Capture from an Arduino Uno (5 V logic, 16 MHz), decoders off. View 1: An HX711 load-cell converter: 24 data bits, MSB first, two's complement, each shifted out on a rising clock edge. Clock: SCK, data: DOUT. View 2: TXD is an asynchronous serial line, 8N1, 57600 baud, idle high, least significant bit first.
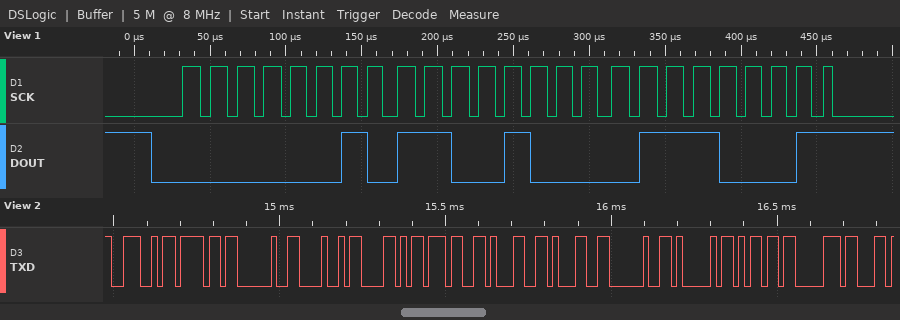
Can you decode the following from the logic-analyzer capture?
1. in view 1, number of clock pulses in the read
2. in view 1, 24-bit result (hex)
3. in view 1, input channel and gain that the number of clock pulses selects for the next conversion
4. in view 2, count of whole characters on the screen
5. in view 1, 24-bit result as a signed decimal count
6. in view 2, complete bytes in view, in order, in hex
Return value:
25
0x02C871
channel A, gain 128
12
182385
0x4E 0x6F 0x20 0x48 0x58 0x37 0x31 0x31 0x20 0x41 0x6D 0x70
